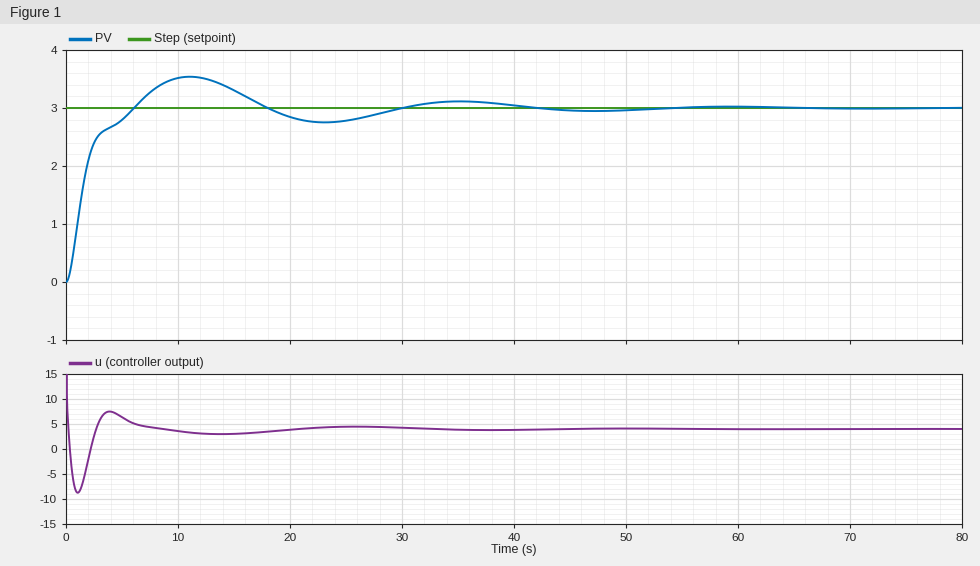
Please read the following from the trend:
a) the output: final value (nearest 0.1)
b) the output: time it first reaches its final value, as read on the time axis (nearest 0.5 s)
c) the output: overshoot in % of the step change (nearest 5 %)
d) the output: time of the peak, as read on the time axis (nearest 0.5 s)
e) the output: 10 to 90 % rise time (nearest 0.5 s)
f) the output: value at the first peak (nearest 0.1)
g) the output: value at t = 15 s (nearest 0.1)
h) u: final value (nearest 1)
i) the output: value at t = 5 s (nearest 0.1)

3.0
6.0 s
20 %
11.0 s
4.0 s
3.5
3.3
4
2.8
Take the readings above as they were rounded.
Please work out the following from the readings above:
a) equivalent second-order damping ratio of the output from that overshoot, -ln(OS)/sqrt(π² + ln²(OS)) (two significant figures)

0.46
